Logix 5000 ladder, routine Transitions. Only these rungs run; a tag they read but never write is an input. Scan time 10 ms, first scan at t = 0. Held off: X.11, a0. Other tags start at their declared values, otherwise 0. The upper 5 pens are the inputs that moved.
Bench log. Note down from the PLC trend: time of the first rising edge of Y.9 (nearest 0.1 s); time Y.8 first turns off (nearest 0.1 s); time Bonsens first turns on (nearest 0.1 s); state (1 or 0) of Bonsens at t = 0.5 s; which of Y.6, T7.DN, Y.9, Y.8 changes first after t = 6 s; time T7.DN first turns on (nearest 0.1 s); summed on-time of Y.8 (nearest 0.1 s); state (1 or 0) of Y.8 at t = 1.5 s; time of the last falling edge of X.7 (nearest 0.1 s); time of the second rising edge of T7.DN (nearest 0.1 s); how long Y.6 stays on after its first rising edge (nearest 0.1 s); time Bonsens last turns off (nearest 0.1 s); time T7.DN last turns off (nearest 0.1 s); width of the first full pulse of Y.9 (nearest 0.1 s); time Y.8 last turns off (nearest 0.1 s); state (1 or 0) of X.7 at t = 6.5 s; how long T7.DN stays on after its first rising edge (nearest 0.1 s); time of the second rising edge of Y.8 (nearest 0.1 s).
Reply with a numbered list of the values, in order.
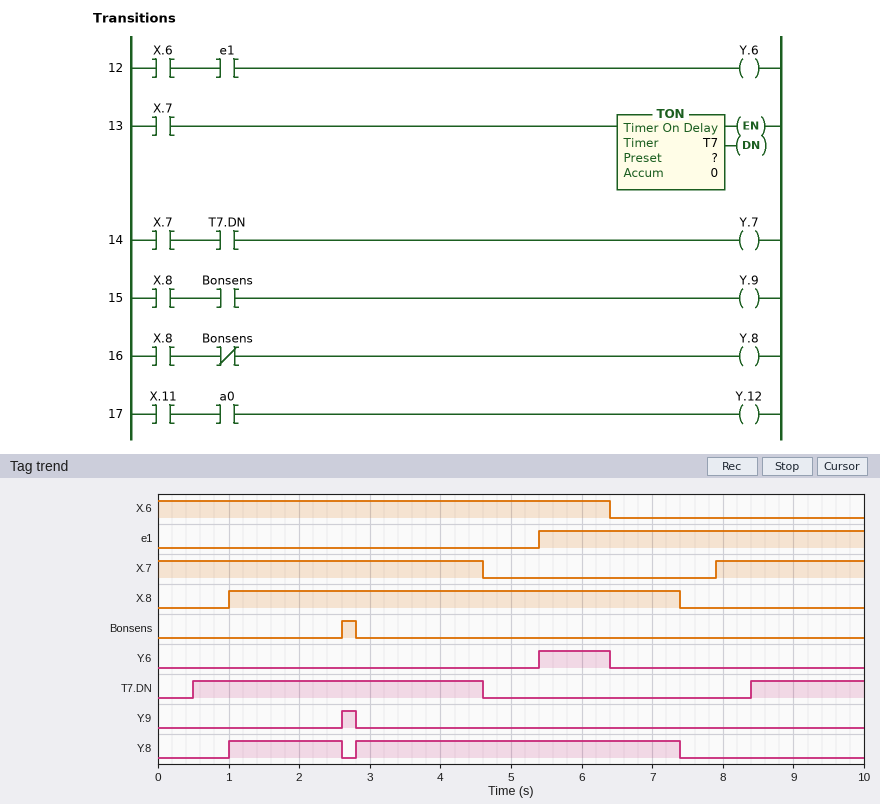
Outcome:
1. 2.6 s
2. 2.6 s
3. 2.6 s
4. 0
5. Y.6
6. 0.5 s
7. 6.2 s
8. 1
9. 4.6 s
10. 8.4 s
11. 1.0 s
12. 2.8 s
13. 4.6 s
14. 0.2 s
15. 7.4 s
16. 0
17. 4.1 s
18. 2.8 s
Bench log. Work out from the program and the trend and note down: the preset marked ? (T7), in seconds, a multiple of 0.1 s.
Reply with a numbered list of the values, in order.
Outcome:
1. 0.5 s
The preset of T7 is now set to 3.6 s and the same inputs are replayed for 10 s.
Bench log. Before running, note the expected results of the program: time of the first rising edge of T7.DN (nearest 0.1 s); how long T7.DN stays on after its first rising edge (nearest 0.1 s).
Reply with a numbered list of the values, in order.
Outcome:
1. 3.6 s
2. 1.0 s
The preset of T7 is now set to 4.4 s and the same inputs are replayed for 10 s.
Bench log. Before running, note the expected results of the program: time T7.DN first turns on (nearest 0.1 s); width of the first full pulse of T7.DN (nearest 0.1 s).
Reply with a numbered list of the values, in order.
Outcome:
1. 4.4 s
2. 0.2 s
